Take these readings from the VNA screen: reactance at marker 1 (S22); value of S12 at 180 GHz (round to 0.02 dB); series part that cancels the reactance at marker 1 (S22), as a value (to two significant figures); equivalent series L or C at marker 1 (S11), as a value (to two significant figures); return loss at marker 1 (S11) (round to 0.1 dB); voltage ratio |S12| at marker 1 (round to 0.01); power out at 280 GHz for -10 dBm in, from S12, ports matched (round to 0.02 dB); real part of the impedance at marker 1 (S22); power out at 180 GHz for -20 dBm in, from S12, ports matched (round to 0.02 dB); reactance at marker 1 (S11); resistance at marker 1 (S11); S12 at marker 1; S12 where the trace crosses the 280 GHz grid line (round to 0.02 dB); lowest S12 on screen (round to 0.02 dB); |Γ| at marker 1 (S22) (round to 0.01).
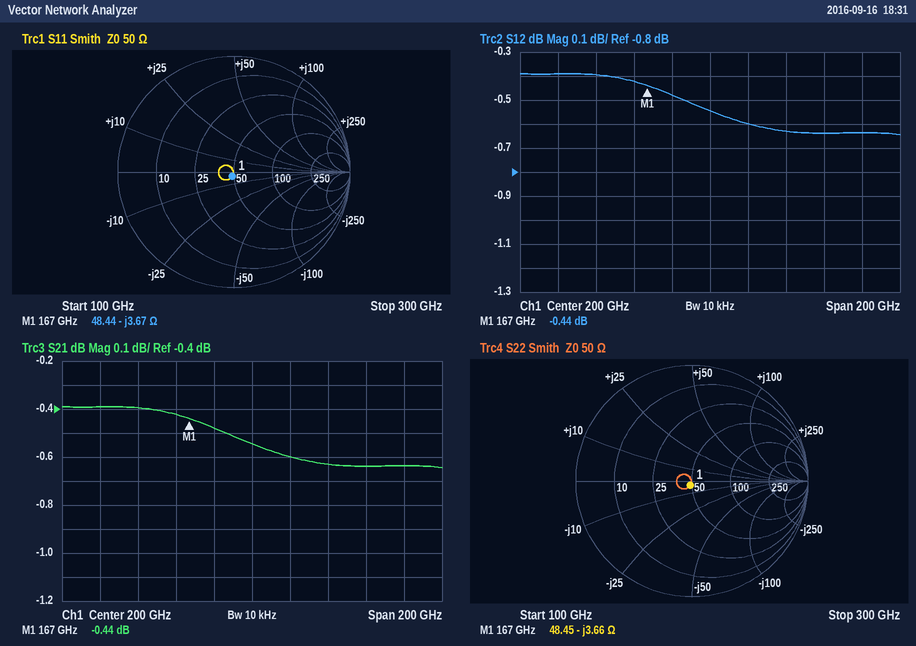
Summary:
-3.66 Ω
-0.48 dB
3.5 pH
260 fF
27.9 dB
0.95
-10.64 dBm
48.45 Ω
-20.48 dBm
-3.67 Ω
48.44 Ω
-0.44 dB
-0.64 dB
-0.64 dB
0.04
